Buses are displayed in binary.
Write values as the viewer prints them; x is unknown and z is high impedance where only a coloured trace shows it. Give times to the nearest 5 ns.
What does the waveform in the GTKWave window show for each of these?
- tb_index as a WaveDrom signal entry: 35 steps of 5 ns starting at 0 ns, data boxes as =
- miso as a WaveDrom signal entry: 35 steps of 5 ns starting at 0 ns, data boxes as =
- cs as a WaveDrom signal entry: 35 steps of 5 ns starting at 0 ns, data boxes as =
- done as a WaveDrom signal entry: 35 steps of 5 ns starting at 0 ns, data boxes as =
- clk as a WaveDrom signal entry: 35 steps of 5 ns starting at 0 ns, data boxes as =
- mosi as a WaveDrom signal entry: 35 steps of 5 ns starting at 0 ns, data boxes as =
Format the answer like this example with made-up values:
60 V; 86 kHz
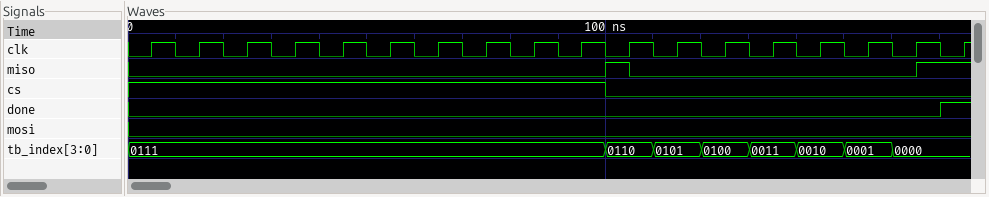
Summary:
{name: 'tb_index', wave: '=...................=.=.=.=.=.=.=..', data: '0111 0110 0101 0100 0011 0010 0001 0000'}; {name: 'miso', wave: '0...................10...........1.'}; {name: 'cs', wave: '1...................0..............'}; {name: 'done', wave: '0.................................1'}; {name: 'clk', wave: '01010101010101010101010101010101010'}; {name: 'mosi', wave: '0..................................'}
